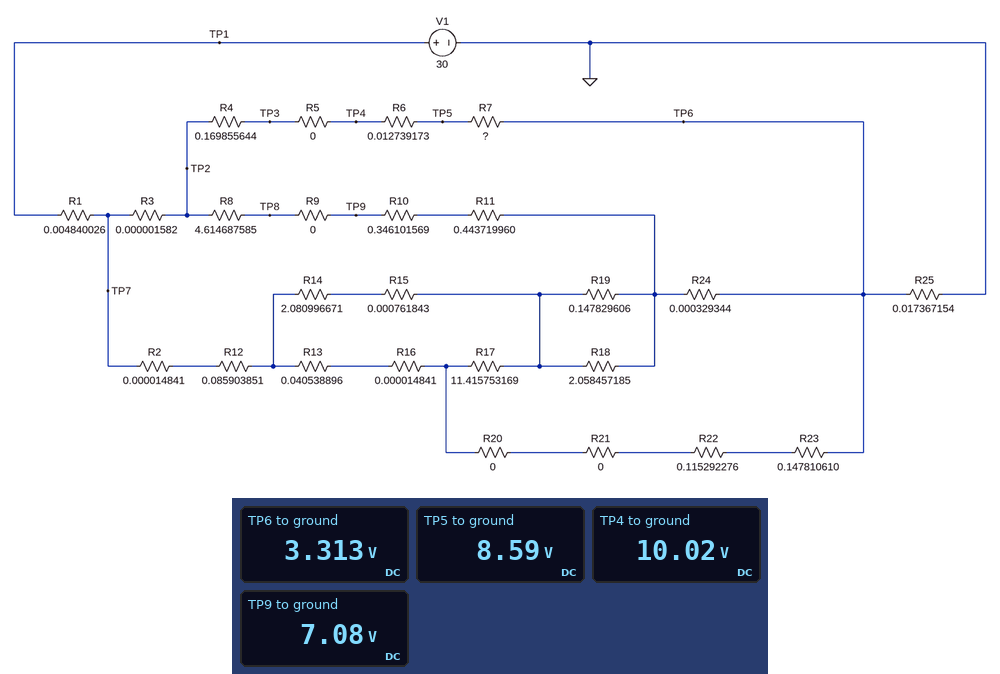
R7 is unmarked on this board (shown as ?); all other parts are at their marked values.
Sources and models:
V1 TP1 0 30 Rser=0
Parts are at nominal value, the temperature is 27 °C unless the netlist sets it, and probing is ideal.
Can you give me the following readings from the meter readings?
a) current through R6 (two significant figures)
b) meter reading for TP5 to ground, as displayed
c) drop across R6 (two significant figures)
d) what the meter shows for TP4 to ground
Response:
110 A
8.59 V
1.4 V
10.02 V
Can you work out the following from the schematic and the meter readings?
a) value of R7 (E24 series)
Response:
0.047 Ω
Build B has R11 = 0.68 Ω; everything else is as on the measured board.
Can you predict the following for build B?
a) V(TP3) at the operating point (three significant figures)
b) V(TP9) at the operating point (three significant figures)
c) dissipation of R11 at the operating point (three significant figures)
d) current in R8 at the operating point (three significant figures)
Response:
10.0 V
8.00 V
14.2 W
4.57 A
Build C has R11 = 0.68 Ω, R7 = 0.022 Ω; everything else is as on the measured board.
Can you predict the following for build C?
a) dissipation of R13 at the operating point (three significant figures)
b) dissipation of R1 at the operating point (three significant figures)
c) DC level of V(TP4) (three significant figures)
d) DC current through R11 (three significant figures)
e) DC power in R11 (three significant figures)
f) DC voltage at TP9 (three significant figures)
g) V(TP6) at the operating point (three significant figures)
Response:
169 W
198 W
7.84 V
4.52 A
13.9 W
8.16 V
3.51 V
